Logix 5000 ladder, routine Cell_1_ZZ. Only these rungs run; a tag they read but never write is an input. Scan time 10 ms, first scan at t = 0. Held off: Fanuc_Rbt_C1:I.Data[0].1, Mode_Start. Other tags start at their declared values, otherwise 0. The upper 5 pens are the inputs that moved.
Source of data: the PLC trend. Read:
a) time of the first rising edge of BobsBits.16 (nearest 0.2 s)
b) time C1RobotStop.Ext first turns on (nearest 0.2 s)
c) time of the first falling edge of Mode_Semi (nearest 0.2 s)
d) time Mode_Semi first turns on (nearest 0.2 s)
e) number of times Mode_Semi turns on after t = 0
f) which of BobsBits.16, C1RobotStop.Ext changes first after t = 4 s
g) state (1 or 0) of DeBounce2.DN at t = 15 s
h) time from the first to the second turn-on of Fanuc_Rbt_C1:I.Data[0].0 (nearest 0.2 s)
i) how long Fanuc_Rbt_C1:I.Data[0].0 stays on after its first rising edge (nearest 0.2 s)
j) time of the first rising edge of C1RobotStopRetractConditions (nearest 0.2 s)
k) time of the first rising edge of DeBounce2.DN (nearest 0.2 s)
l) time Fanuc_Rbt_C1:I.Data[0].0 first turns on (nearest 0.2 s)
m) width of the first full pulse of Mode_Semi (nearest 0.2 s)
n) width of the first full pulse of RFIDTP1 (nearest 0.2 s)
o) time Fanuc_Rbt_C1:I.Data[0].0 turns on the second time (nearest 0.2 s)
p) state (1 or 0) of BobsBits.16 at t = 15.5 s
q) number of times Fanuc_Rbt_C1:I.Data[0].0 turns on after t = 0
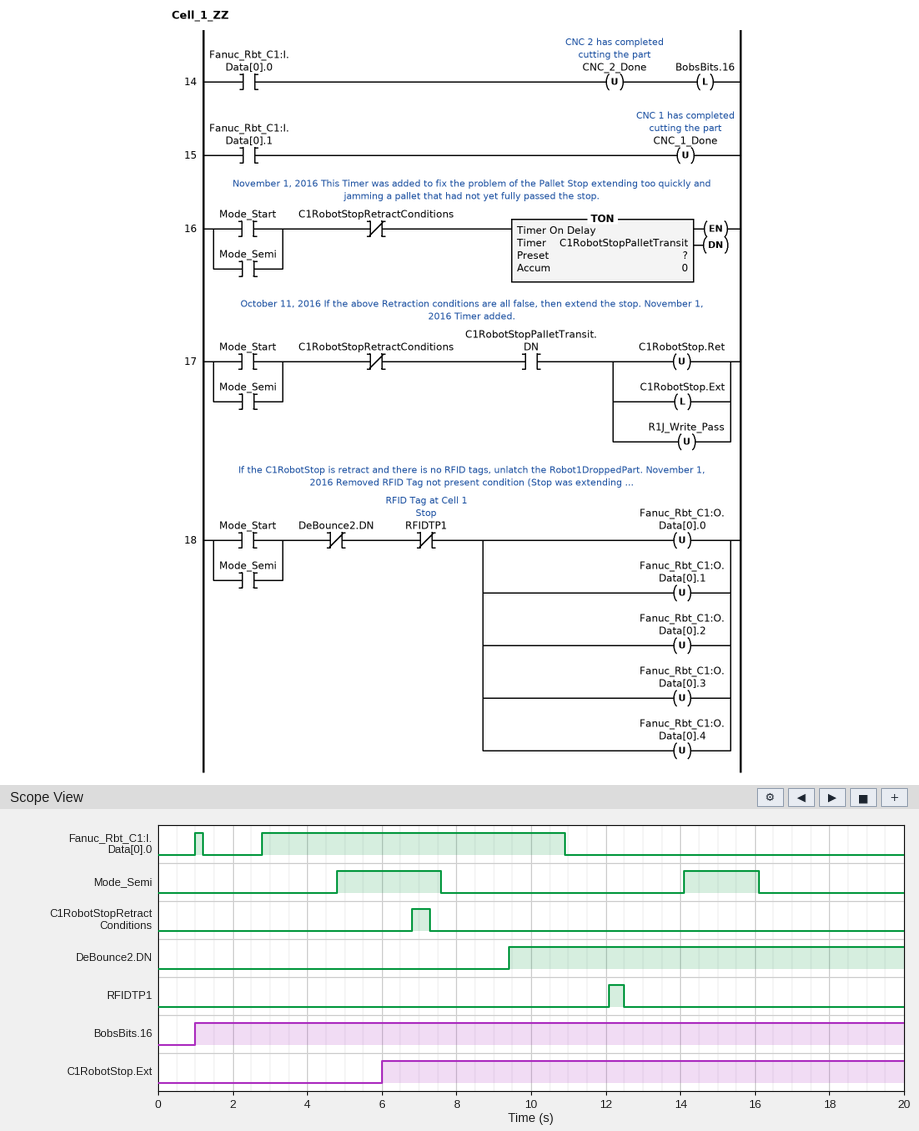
1.0 s
6.0 s
7.6 s
4.8 s
2
C1RobotStop.Ext
1
1.8 s
0.2 s
6.8 s
9.4 s
1.0 s
2.8 s
0.4 s
2.8 s
1
2
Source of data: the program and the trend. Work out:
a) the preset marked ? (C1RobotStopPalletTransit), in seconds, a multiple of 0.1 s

1.2 s
